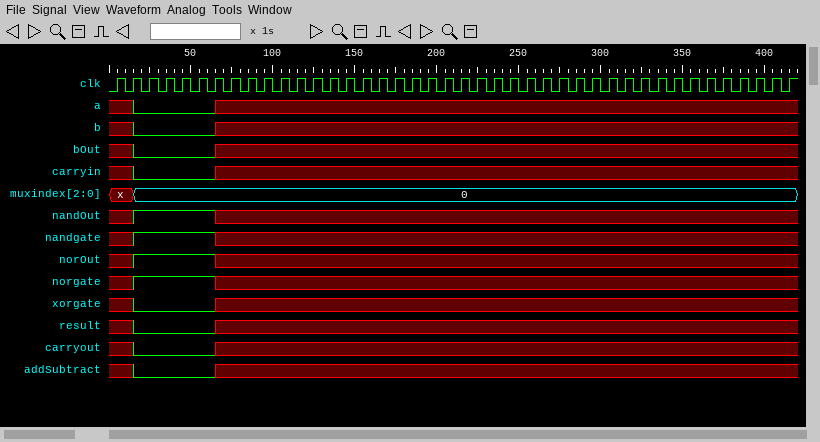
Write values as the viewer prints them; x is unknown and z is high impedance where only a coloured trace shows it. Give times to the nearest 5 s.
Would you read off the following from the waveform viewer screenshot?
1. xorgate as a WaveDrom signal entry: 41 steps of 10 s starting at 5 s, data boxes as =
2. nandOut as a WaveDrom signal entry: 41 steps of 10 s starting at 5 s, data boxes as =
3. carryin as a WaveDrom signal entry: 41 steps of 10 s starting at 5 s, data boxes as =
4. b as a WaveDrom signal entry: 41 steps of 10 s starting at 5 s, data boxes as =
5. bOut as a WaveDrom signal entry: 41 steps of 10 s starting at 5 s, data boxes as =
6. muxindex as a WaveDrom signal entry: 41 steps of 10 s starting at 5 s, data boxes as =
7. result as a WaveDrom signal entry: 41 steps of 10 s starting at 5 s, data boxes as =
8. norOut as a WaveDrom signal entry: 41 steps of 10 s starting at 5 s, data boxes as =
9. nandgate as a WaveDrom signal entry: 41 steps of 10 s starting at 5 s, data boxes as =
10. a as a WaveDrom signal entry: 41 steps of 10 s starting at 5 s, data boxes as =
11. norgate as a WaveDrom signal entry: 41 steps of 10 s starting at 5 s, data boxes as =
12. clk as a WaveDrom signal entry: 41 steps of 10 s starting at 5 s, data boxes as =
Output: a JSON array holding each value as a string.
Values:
["{name: 'xorgate', wave: 'x0....x..................................'}", "{name: 'nandOut', wave: 'x1....x..................................'}", "{name: 'carryin', wave: 'x0....x..................................'}", "{name: 'b', wave: 'x0....x..................................'}", "{name: 'bOut', wave: 'x0....x..................................'}", "{name: 'muxindex', wave: 'x=.......................................', data: '0'}", "{name: 'result', wave: 'x0....x..................................'}", "{name: 'norOut', wave: 'x1....x..................................'}", "{name: 'nandgate', wave: 'x1....x..................................'}", "{name: 'a', wave: 'x0....x..................................'}", "{name: 'norgate', wave: 'x1....x..................................'}", "{name: 'clk', wave: 'p........................................'}"]
